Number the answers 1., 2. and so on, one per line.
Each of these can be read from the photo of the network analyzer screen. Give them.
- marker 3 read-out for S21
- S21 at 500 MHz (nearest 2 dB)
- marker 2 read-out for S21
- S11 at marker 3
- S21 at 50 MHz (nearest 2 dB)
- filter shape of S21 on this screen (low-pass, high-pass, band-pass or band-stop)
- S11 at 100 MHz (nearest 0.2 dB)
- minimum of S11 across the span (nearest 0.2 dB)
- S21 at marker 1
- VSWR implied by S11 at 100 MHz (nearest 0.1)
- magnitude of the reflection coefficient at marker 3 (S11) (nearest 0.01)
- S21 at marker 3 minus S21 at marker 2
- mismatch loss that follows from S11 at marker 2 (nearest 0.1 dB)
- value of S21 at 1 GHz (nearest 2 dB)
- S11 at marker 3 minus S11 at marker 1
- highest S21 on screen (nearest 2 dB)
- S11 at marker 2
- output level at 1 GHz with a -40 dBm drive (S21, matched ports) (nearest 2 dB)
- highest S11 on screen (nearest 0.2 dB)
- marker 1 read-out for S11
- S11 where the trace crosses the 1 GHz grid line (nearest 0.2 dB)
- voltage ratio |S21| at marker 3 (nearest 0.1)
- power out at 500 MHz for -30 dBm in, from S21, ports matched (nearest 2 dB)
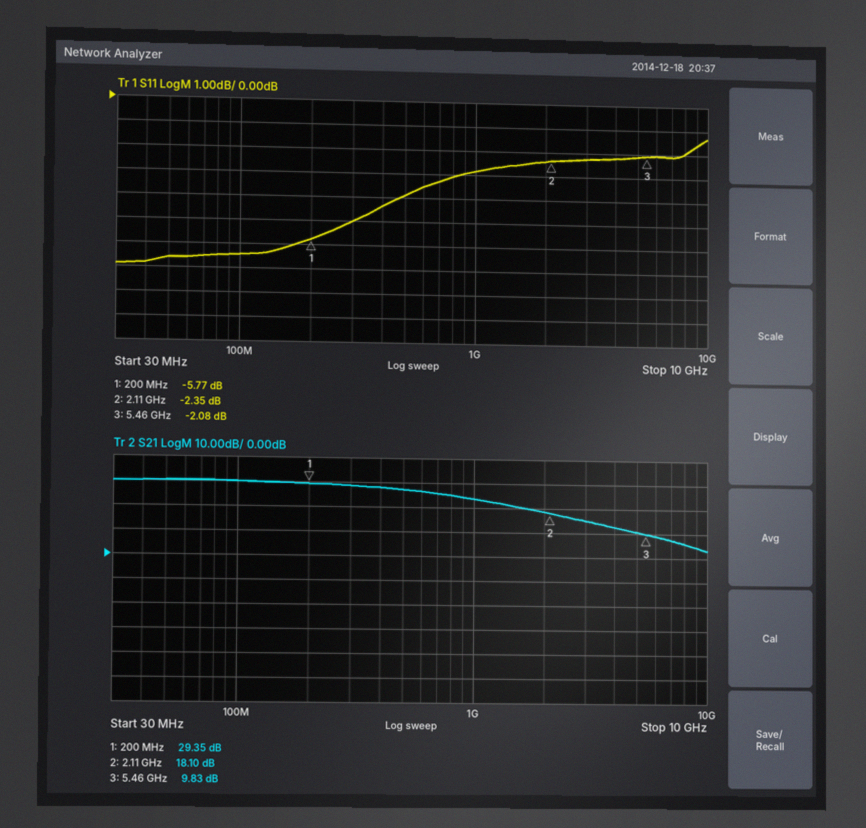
1. 9.83 dB
2. 28 dB
3. 18.10 dB
4. -2.08 dB
5. 30 dB
6. low-pass
7. -6.4 dB
8. -6.8 dB
9. 29.35 dB
10. 2.8
11. 0.79
12. -8.27 dB
13. 3.8 dB
14. 24 dB
15. 3.69 dB
16. 30 dB
17. -2.35 dB
18. -16 dBm
19. -1.4 dB
20. -5.77 dB
21. -2.8 dB
22. 3.1
23. -2 dBm
